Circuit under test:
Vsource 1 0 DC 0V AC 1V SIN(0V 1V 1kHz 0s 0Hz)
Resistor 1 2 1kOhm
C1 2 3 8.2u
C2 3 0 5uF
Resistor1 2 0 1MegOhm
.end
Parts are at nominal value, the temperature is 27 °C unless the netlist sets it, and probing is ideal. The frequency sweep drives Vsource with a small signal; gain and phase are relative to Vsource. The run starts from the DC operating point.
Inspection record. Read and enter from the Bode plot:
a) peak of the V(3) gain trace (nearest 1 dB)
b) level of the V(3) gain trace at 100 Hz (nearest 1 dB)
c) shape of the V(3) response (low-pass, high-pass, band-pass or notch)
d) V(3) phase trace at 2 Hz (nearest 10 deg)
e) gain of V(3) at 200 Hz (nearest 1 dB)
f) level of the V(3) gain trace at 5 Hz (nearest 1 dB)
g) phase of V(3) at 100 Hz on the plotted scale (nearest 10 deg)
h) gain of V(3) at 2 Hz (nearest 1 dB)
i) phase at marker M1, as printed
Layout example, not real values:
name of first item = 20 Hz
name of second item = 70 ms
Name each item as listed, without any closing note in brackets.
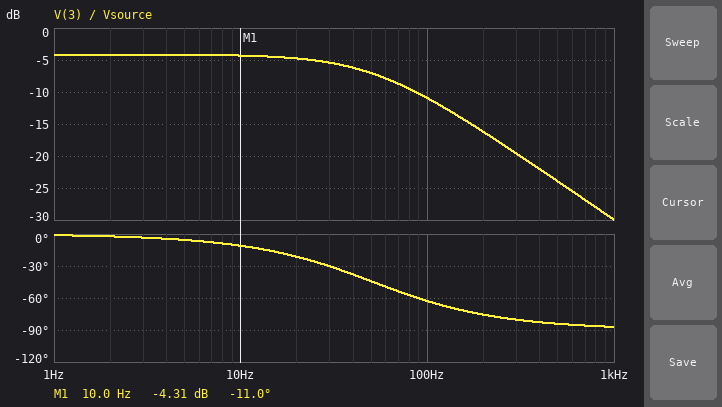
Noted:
peak of the V(3) gain trace = -4 dB
level of the V(3) gain trace at 100 Hz = -11 dB
shape of the V(3) response = low-pass
V(3) phase trace at 2 Hz = 0 deg
gain of V(3) at 200 Hz = -16 dB
level of the V(3) gain trace at 5 Hz = -4 dB
phase of V(3) at 100 Hz on the plotted scale = -60 deg
gain of V(3) at 2 Hz = -4 dB
phase at marker M1, as printed = -11.0 deg
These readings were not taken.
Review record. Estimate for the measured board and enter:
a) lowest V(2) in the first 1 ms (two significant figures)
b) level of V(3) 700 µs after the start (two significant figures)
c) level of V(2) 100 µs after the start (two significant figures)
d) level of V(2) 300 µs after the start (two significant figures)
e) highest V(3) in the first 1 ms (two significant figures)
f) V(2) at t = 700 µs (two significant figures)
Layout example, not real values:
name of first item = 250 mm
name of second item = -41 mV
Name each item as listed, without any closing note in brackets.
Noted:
lowest V(2) in the first 1 ms = -14 mV
level of V(3) 700 µs after the start = 34 mV
level of V(2) 100 µs after the start = 9.7 mV
level of V(2) 300 µs after the start = 65 mV
highest V(3) in the first 1 ms = 59 mV
V(2) at t = 700 µs = 54 mV
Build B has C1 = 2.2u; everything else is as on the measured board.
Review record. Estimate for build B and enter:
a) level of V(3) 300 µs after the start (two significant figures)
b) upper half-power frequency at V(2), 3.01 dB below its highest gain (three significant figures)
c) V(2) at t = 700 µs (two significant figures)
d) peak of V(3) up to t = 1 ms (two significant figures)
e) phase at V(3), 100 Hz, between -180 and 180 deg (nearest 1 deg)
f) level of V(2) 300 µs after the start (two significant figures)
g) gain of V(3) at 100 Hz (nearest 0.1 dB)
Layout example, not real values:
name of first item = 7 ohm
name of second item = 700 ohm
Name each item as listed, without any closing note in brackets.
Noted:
level of V(3) 300 µs after the start = 39 mV
upper half-power frequency at V(2), 3.01 dB below its highest gain = 104 Hz
V(2) at t = 700 µs = 87 mV
peak of V(3) up to t = 1 ms = 55 mV
phase at V(3), 100 Hz, between -180 and 180 deg = -44 deg
level of V(2) 300 µs after the start = 130 mV
gain of V(3) at 100 Hz = -13.1 dB
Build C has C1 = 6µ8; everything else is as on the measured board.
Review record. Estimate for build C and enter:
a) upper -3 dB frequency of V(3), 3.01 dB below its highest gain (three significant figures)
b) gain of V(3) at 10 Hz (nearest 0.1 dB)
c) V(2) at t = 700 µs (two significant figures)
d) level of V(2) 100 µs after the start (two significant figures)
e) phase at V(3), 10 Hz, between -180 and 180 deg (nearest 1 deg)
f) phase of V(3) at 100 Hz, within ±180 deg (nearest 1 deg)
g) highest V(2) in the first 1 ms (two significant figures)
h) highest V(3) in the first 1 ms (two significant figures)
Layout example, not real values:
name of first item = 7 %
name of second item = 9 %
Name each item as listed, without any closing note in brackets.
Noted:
upper -3 dB frequency of V(3), 3.01 dB below its highest gain = 55.3 Hz
gain of V(3) at 10 Hz = -4.9 dB
V(2) at t = 700 µs = 57 mV
level of V(2) 100 µs after the start = 10 mV
phase at V(3), 10 Hz, between -180 and 180 deg = -10 deg
phase of V(3) at 100 Hz, within ±180 deg = -61 deg
highest V(2) in the first 1 ms = 100 mV
highest V(3) in the first 1 ms = 59 mV
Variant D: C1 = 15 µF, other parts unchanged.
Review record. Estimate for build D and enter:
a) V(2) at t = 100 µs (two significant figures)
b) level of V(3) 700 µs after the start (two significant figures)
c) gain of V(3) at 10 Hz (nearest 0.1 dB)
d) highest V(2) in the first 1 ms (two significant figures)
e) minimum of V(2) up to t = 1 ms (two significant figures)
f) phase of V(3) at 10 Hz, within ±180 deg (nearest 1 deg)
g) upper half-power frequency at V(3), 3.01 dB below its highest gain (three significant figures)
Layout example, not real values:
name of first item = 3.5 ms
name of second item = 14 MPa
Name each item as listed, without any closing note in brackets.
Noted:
V(2) at t = 100 µs = 8.0 mV
level of V(3) 700 µs after the start = 35 mV
gain of V(3) at 10 Hz = -2.7 dB
highest V(2) in the first 1 ms = 80 mV
minimum of V(2) up to t = 1 ms = -9.9 mV
phase of V(3) at 10 Hz, within ±180 deg = -13 deg
upper half-power frequency at V(3), 3.01 dB below its highest gain = 42.5 Hz
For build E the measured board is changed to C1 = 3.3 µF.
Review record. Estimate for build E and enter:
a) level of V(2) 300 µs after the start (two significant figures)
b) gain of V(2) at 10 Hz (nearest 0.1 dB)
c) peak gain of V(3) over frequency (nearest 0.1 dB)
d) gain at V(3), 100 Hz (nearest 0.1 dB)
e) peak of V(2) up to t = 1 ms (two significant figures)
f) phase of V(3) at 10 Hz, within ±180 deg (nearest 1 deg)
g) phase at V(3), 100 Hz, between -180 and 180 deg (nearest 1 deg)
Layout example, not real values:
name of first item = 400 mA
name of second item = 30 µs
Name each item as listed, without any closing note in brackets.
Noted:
level of V(2) 300 µs after the start = 99 mV
gain of V(2) at 10 Hz = -0.1 dB
peak gain of V(3) over frequency = -8.0 dB
gain at V(3), 100 Hz = -12.1 dB
peak of V(2) up to t = 1 ms = 140 mV
phase of V(3) at 10 Hz, within ±180 deg = -7 deg
phase at V(3), 100 Hz, between -180 and 180 deg = -51 deg
